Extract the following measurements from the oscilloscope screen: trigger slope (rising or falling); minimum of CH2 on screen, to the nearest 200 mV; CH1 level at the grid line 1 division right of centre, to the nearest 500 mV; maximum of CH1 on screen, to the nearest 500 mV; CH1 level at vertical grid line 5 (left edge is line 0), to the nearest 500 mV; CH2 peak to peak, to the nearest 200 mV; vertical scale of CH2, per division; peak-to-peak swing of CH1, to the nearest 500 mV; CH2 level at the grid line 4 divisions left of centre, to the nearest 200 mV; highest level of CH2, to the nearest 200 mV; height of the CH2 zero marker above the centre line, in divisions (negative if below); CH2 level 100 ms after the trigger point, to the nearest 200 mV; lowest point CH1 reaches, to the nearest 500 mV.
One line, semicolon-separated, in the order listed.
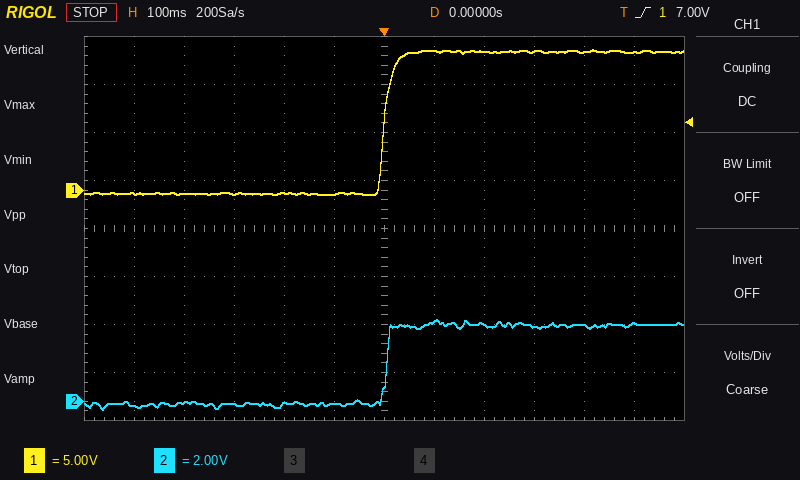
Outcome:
rising; -400 mV; 14.5 V; 14.5 V; -500 mV; 3.8 V; 2 V; 15.0 V; 0.0 V; 3.4 V; -3.6 div; 3.4 V; -500 mV
